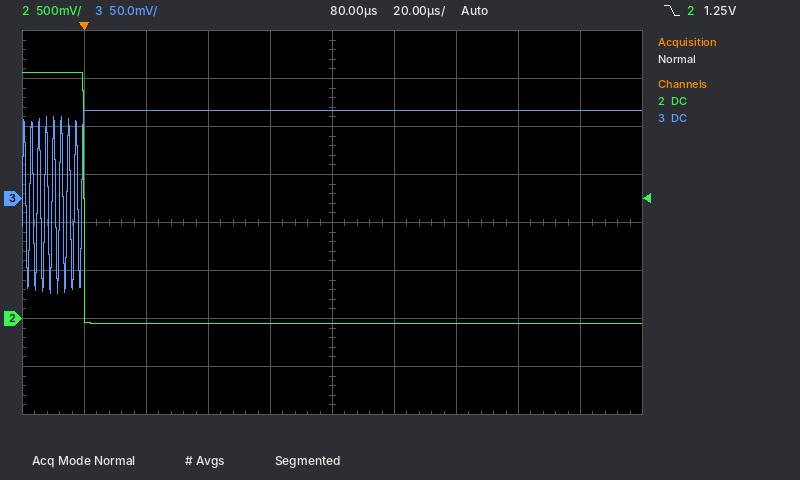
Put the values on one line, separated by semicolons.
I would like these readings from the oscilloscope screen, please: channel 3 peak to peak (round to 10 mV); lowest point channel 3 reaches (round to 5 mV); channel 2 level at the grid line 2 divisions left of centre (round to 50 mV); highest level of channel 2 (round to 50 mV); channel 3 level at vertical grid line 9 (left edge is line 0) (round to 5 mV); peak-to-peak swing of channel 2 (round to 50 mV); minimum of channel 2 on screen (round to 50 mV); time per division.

190 mV; -100 mV; -50 mV; 2.55 V; 90 mV; 2.60 V; -50 mV; 20 µs
